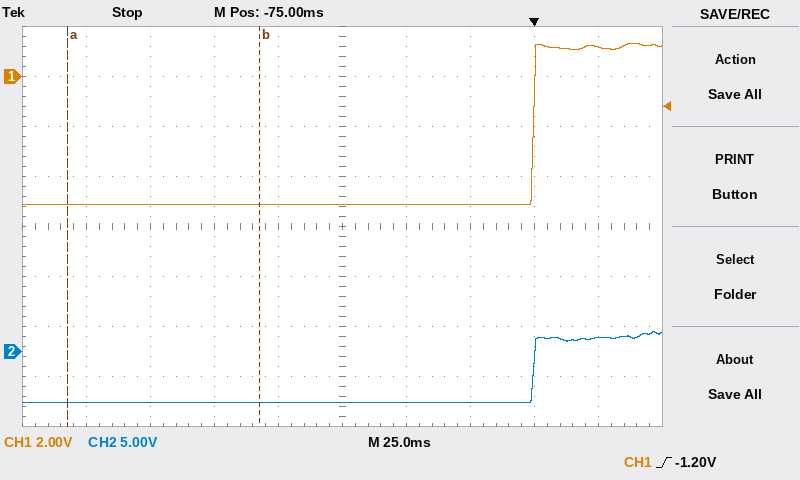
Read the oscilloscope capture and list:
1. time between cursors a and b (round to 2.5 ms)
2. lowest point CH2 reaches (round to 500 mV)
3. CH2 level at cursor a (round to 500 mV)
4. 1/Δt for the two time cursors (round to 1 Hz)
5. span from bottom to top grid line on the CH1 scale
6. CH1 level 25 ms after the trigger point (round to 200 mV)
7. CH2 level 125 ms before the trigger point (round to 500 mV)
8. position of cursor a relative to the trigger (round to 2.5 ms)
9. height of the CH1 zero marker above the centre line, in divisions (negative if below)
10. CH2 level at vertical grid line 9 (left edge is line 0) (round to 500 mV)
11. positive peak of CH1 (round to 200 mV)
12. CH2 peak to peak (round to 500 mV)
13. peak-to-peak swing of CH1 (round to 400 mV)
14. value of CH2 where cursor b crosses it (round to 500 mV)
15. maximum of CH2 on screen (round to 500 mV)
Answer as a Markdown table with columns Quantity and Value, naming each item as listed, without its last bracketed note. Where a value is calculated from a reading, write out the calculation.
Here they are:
| Quantity | Value |
|---|---|
| time between cursors a and b | 75.0 ms |
| lowest point CH2 reaches | -5.0 V |
| CH2 level at cursor a | -5.0 V |
| 1/Δt for the two time cursors | 1 / 75.0 ms ≈ 13 Hz |
| span from bottom to top grid line on the CH1 scale | 16 V |
| CH1 level 25 ms after the trigger point | 1.2 V |
| CH2 level 125 ms before the trigger point | -5.0 V |
| position of cursor a relative to the trigger | -182.5 ms |
| height of the CH1 zero marker above the centre line, in divisions | +3.0 div |
| CH2 level at vertical grid line 9 (left edge is line 0) | 1.5 V |
| positive peak of CH1 | 1.4 V |
| CH2 peak to peak | 2.0 V − (-5.0 V) = 7.0 V |
| peak-to-peak swing of CH1 | 6.4 V |
| value of CH2 where cursor b crosses it | -5.0 V |
| maximum of CH2 on screen | 2.0 V |
